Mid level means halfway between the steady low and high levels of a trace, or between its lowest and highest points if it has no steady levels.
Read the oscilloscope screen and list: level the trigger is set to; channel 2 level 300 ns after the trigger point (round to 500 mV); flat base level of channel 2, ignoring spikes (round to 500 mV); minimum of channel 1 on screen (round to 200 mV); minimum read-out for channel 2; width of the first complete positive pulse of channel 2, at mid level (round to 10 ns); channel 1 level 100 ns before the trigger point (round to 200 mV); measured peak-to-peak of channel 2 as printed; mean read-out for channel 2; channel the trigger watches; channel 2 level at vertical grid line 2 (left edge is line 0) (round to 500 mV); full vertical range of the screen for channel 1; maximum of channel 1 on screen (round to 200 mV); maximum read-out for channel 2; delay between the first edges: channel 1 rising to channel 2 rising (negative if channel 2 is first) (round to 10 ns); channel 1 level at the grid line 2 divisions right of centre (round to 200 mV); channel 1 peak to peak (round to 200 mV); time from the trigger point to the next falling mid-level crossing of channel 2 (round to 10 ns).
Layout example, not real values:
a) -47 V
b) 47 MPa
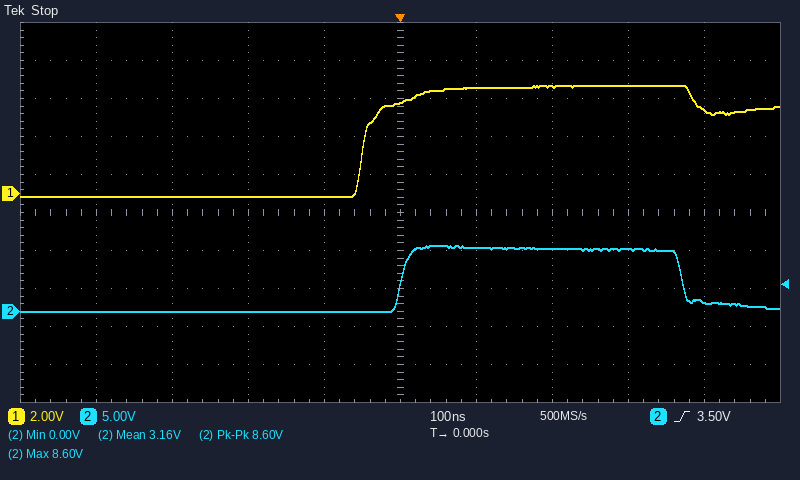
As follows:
a) 3.50 V
b) 8.0 V
c) 0.0 V
d) -200 mV
e) 0.00 V
f) 370 ns
g) -200 mV
h) 8.60 V
i) 3.16 V
j) channel 2
k) 0.0 V
l) 20 V
m) 5.6 V
n) 8.60 V
o) +50 ns
p) 5.6 V
q) 5.8 V
r) 370 ns
